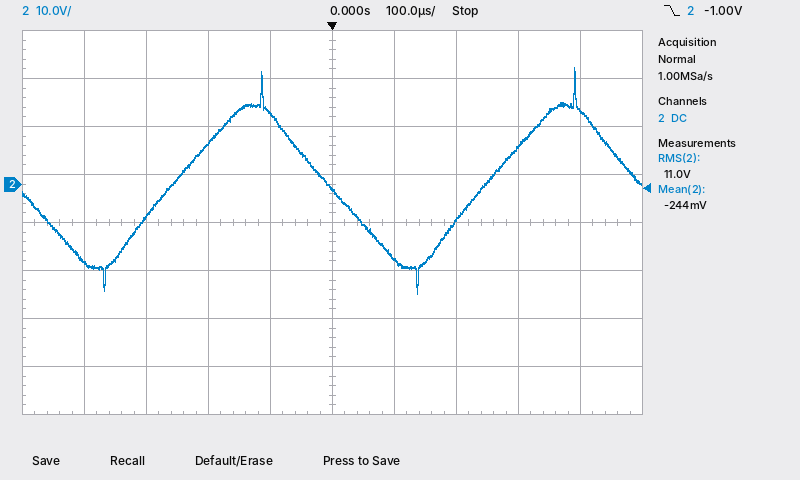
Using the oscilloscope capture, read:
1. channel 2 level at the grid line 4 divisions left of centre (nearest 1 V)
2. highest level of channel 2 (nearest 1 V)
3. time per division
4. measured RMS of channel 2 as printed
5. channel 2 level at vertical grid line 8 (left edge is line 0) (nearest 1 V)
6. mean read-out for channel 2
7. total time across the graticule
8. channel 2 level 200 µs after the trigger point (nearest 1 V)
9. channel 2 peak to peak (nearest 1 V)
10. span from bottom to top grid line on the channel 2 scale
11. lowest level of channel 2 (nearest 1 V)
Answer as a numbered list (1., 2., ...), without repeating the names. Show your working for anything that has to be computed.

1. -16 V
2. 24 V
3. 100 µs
4. 11.0 V
5. 8 V
6. -244 mV
7. 1 ms
8. -8 V
9. 24 V − (-23 V) = 47 V
10. 80 V
11. -23 V
